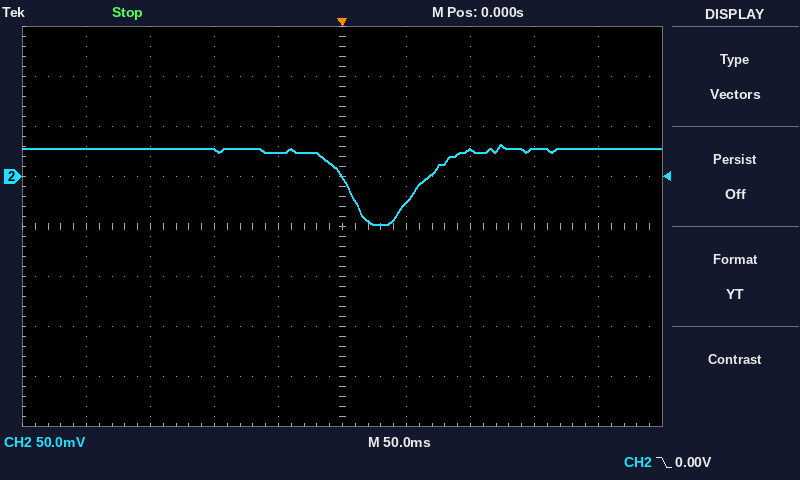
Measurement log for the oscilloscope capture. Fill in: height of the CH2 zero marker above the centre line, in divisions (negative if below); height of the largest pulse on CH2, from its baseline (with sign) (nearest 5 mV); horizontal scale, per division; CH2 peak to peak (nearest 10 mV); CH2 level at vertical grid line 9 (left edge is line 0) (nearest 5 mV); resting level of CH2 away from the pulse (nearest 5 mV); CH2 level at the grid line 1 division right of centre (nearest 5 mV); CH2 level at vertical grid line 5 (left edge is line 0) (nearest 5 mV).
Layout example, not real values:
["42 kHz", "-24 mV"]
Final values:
["+1.0 div", "-75 mV", "50 ms", "80 mV", "30 mV", "30 mV", "-25 mV", "0 mV"]
